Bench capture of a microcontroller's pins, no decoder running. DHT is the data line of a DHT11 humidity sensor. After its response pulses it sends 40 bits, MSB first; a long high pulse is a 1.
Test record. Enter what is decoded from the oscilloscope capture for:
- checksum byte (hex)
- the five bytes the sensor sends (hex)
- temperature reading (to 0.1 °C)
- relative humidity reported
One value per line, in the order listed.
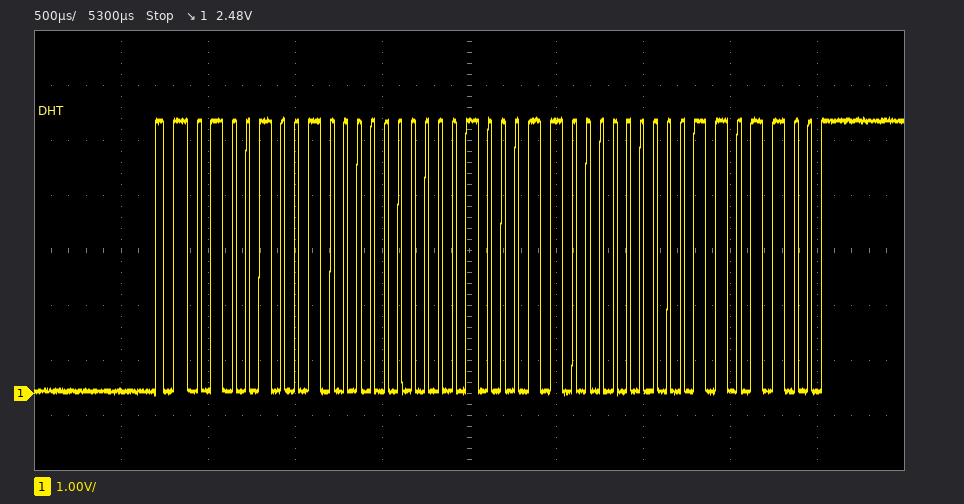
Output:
0x6C
49 00 23 00 6C
35.0 °C
73 %
